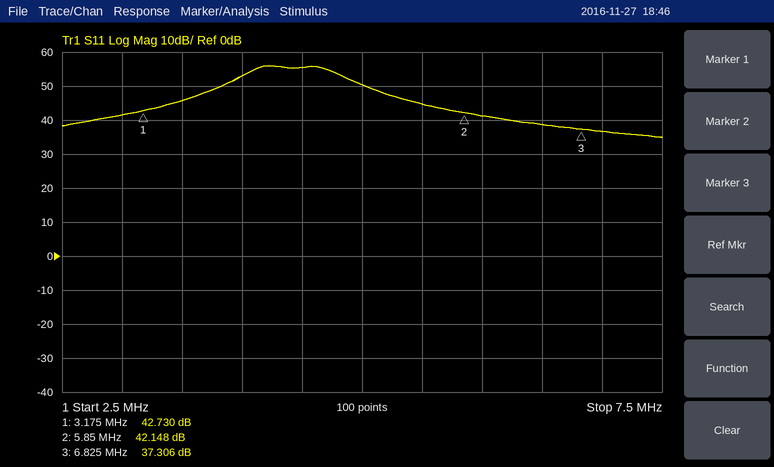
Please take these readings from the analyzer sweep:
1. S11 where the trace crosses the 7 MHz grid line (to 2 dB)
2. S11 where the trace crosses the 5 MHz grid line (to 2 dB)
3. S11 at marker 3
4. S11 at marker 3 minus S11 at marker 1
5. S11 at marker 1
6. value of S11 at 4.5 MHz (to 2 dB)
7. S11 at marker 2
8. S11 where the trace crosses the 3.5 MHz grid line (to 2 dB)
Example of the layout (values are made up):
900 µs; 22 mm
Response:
36 dB; 50 dB; 37.306 dB; -5.424 dB; 42.730 dB; 56 dB; 42.148 dB; 46 dB
